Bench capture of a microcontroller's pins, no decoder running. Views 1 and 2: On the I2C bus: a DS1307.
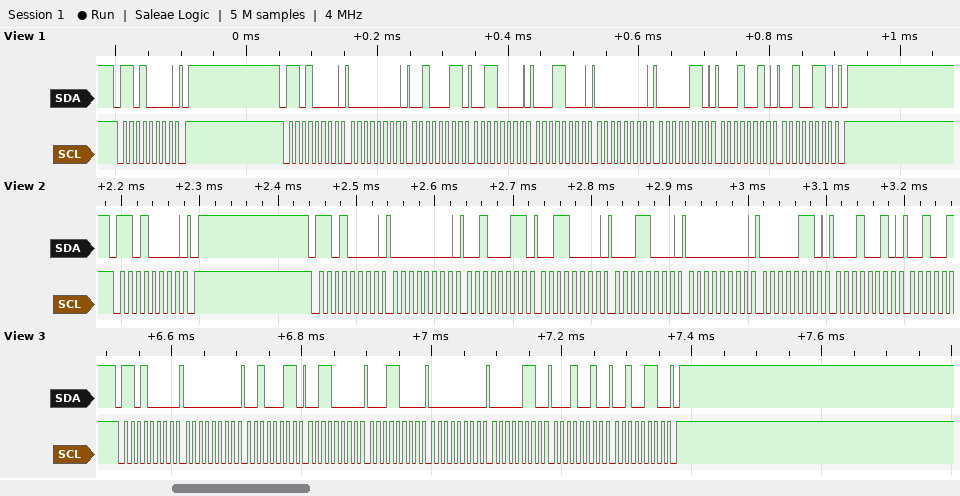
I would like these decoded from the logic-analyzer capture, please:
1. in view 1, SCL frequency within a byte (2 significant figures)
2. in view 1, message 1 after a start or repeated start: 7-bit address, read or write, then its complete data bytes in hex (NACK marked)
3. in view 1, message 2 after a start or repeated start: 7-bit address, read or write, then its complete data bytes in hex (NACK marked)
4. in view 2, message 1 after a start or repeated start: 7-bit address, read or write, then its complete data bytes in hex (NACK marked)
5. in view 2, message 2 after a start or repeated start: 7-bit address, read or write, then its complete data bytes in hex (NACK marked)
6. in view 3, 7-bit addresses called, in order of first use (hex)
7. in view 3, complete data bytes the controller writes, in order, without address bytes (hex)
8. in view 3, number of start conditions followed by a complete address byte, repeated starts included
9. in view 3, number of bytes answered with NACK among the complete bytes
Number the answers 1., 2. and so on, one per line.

1. 100 kHz
2. 0x68 write
3. 0x68 write: 00 23 30 18 00 06 12 26
4. 0x68 write
5. 0x68 write: 00 23 30 18 00 06 12
6. 0x68
7. 00 23 30 18 00 06 12 26
8. 1
9. 0
